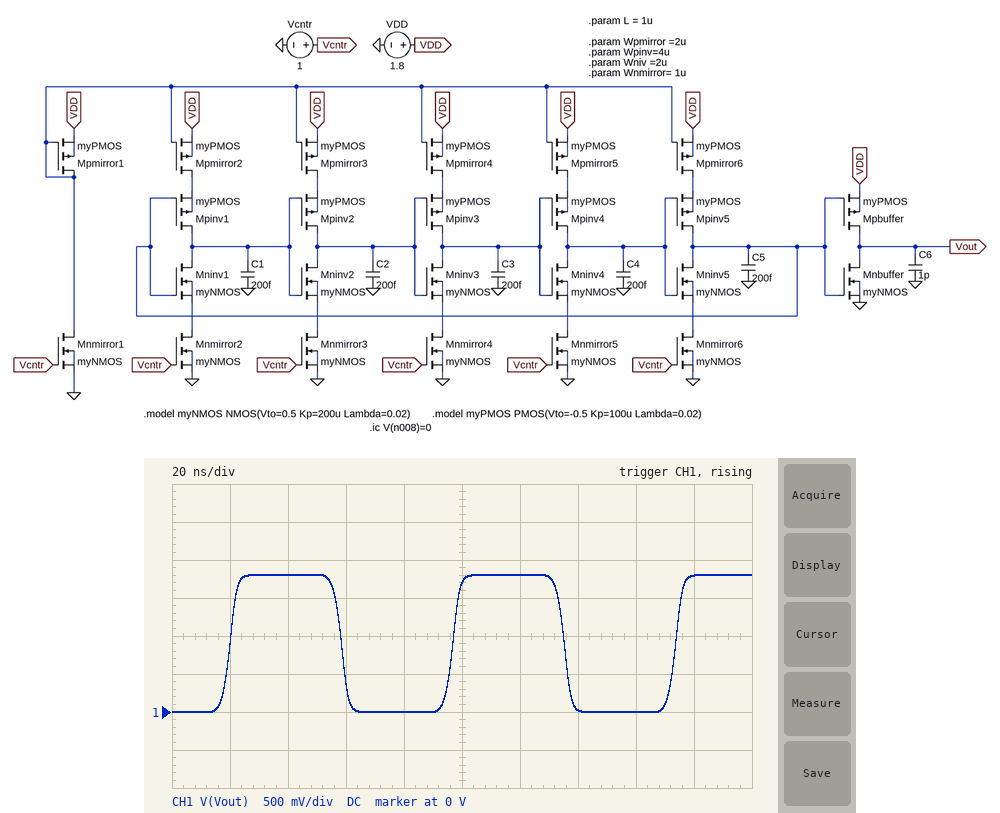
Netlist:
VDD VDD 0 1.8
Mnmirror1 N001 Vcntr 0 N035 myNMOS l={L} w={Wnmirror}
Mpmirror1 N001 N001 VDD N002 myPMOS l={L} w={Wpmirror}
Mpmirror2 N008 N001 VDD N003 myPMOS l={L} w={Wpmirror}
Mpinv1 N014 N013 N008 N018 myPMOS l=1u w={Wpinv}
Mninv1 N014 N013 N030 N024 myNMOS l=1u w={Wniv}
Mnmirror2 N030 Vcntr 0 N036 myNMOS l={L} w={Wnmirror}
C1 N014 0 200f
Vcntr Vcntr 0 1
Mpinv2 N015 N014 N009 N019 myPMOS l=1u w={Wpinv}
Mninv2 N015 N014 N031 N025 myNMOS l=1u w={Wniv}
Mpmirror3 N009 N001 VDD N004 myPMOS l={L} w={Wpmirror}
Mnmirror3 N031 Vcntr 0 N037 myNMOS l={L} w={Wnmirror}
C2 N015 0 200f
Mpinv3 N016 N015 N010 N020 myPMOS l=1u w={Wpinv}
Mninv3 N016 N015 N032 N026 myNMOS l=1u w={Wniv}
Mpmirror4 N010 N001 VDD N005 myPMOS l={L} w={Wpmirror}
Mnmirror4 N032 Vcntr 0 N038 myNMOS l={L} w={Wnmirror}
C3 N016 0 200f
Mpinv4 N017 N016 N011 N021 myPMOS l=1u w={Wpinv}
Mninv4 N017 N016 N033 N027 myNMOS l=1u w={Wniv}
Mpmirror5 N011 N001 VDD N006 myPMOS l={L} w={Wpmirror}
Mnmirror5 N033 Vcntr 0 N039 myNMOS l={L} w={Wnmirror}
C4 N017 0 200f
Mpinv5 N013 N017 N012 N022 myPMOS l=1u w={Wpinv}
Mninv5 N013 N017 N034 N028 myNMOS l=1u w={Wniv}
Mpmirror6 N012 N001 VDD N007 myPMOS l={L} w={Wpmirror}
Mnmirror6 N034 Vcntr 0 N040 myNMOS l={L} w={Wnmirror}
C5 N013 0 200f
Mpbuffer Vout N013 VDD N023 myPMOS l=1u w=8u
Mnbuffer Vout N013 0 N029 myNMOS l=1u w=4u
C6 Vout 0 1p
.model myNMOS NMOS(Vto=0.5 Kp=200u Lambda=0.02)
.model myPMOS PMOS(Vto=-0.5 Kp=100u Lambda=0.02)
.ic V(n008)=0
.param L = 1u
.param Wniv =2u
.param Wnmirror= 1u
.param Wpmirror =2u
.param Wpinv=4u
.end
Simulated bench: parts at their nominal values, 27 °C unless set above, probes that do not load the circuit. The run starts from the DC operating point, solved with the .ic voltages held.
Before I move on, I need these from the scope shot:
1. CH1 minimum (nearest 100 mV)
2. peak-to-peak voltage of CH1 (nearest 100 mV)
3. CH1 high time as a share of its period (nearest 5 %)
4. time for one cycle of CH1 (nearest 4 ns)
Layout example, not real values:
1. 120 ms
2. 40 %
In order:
1. 0 V
2. 1.8 V
3. 50 %
4. 76 ns
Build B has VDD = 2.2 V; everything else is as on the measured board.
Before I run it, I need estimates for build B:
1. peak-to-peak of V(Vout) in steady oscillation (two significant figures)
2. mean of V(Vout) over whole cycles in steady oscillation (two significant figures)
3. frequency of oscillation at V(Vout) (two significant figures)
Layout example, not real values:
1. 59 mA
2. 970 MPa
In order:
1. 2.2 V
2. 1.1 V
3. 11 MHz
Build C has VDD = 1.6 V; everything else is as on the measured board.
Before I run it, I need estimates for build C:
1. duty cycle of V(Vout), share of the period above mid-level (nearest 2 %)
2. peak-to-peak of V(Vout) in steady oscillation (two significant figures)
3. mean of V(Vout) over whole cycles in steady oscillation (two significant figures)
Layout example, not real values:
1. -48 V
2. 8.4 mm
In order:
1. 50 %
2. 1.6 V
3. 800 mV
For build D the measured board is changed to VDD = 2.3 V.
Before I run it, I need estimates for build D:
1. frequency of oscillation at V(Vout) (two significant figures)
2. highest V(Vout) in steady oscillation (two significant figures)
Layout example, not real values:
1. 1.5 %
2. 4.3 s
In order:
1. 11 MHz
2. 2.3 V
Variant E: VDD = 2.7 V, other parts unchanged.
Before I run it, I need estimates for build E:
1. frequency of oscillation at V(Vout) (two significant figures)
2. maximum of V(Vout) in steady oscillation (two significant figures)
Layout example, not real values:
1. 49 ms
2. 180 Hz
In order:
1. 8.8 MHz
2. 2.7 V
